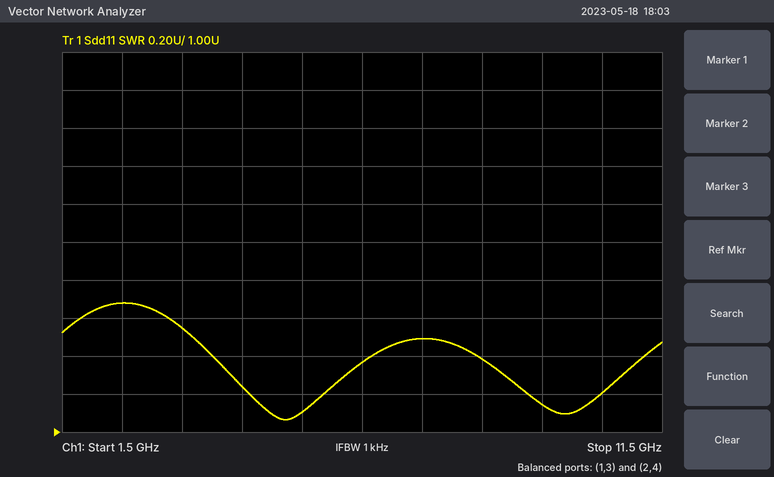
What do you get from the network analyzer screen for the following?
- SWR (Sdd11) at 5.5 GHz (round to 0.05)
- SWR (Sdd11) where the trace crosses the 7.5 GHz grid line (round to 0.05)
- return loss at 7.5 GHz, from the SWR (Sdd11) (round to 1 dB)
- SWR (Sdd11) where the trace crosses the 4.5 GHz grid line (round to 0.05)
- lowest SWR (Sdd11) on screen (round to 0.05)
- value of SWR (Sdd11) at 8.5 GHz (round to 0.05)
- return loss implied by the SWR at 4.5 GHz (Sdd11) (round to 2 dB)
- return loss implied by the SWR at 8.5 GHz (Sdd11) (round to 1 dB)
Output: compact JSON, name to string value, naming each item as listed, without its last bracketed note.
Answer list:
{"SWR (Sdd11) at 5.5 GHz": "1.10", "SWR (Sdd11) where the trace crosses the 7.5 GHz grid line": "1.50", "return loss at 7.5 GHz, from the SWR (Sdd11)": "14 dB", "SWR (Sdd11) where the trace crosses the 4.5 GHz grid line": "1.25", "lowest SWR (Sdd11) on screen": "1.05", "value of SWR (Sdd11) at 8.5 GHz": "1.40", "return loss implied by the SWR at 4.5 GHz (Sdd11)": "20 dB", "return loss implied by the SWR at 8.5 GHz (Sdd11)": "16 dB"}
